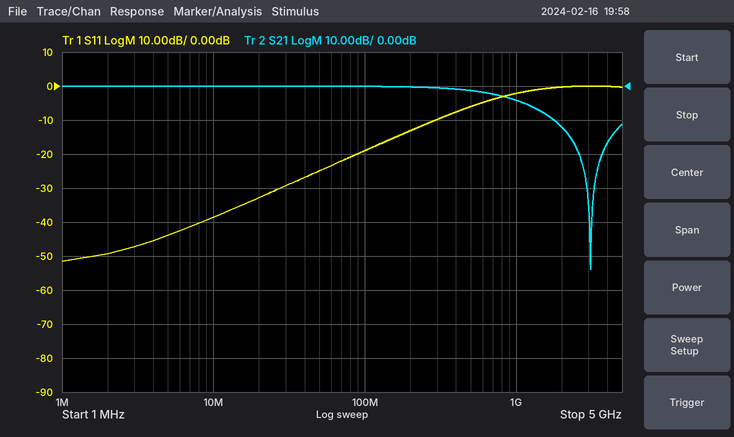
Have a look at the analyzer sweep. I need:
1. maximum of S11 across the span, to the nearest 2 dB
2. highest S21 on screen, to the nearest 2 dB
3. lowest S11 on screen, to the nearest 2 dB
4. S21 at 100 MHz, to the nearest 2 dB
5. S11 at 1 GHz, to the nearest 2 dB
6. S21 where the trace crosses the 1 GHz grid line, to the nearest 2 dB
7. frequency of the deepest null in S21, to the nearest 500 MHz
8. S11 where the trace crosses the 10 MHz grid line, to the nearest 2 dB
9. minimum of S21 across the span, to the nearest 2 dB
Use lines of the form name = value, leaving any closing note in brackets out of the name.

maximum of S11 across the span, to the nearest 2 dB = 0 dB
highest S21 on screen, to the nearest 2 dB = 0 dB
lowest S11 on screen, to the nearest 2 dB = -52 dB
S21 at 100 MHz, to the nearest 2 dB = 0 dB
S11 at 1 GHz, to the nearest 2 dB = -2 dB
S21 where the trace crosses the 1 GHz grid line, to the nearest 2 dB = -4 dB
frequency of the deepest null in S21, to the nearest 500 MHz = 3.0 GHz
S11 where the trace crosses the 10 MHz grid line, to the nearest 2 dB = -38 dB
minimum of S21 across the span, to the nearest 2 dB = -54 dB
